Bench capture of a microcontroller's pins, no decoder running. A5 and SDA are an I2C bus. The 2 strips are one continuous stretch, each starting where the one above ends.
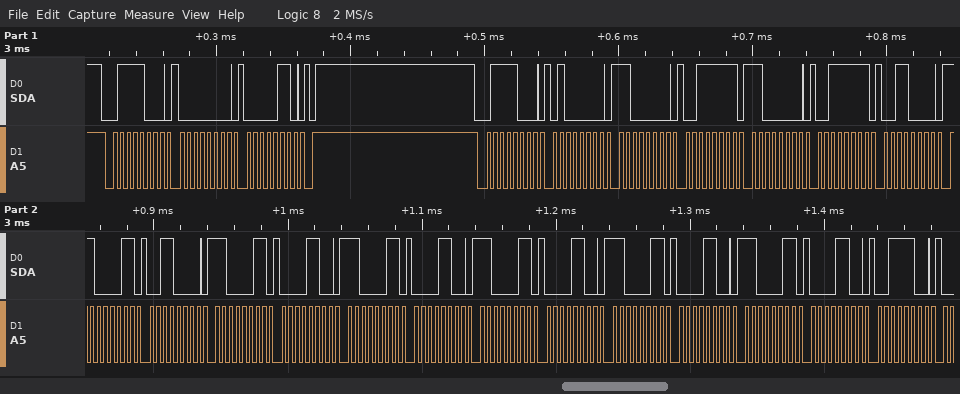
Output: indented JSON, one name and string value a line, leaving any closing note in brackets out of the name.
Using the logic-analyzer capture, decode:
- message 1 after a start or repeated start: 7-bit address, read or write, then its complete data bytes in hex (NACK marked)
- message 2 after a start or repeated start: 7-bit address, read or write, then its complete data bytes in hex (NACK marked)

{
  "message 1 after a start or repeated start: 7-bit address, read or write, then its complete data bytes in hex": "0x3C write: 00 06",
  "message 2 after a start or repeated start: 7-bit address, read or write, then its complete data bytes in hex": "0x3C write: 40 C0 3F C0 3F 30 C3 30 C3 0C C3 0C C3 0C C3 0C C3 0C 3C"
}
